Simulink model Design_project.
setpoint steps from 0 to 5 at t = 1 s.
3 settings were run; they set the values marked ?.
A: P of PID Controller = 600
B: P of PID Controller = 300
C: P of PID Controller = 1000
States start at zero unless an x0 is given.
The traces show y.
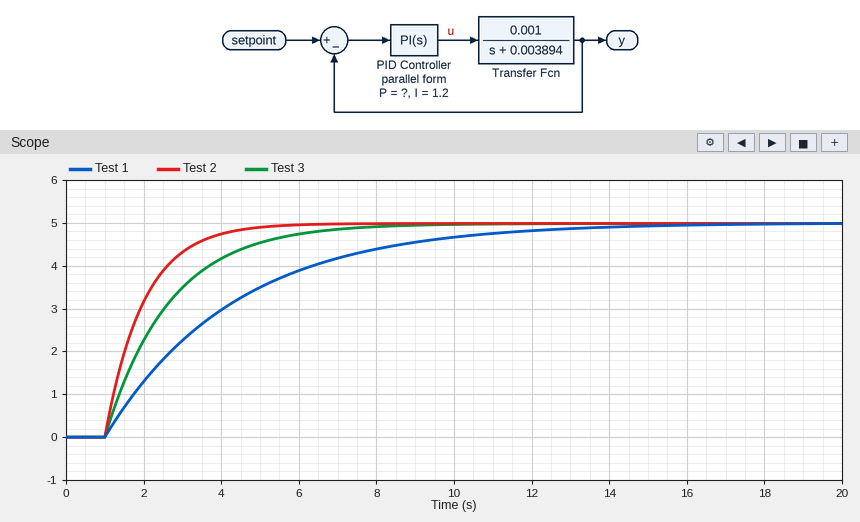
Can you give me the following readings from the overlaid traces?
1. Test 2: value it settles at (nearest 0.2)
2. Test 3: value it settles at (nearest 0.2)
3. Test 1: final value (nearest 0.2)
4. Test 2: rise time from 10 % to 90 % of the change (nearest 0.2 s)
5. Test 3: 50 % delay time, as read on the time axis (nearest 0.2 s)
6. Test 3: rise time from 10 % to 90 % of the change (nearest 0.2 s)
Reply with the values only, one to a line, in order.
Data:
5.0
5.0
5.0
2.2 s
2.2 s
3.6 s
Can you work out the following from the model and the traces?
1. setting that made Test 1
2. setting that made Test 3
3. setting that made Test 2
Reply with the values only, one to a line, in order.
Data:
B
A
C
